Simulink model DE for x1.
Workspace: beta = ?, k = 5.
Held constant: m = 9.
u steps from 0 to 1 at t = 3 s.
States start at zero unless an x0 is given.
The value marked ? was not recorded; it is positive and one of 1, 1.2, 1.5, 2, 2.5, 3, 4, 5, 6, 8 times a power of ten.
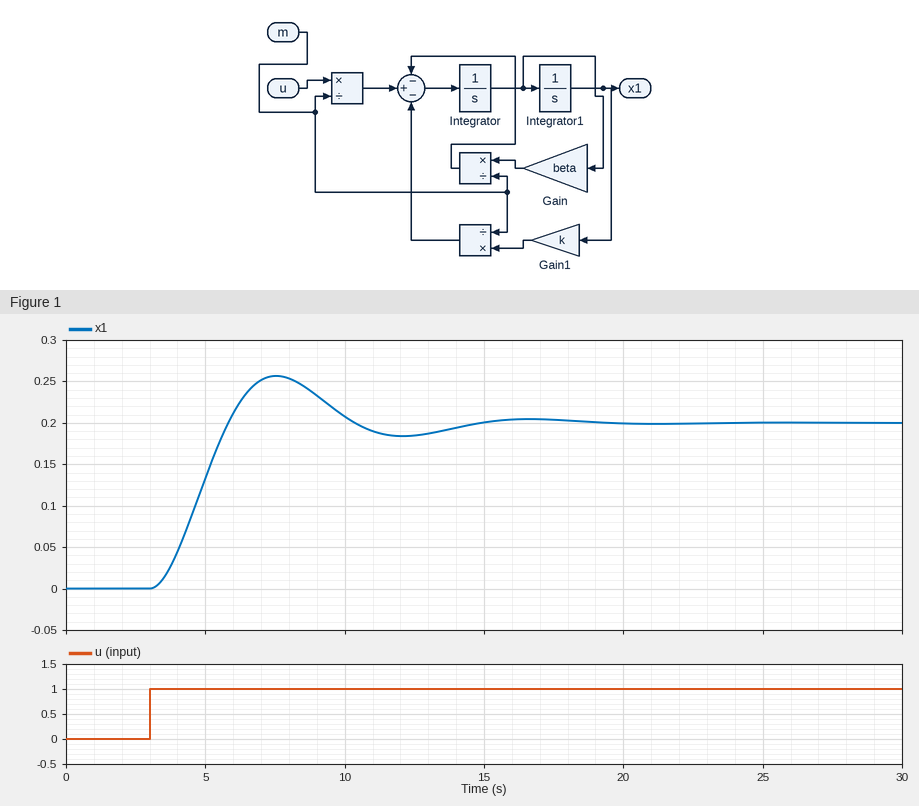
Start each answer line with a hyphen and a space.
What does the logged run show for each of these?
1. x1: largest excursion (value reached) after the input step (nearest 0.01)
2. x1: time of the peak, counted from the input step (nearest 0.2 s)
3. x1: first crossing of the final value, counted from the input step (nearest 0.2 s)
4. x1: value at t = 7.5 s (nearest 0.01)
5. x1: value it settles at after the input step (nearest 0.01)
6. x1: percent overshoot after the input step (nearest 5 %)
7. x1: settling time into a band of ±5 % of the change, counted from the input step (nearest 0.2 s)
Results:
- 0.26
- 4.6 s
- 2.8 s
- 0.26
- 0.20
- 30 %
- 10.4 s
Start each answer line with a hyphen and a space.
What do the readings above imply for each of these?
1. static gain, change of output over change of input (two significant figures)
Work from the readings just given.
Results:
- 0.20
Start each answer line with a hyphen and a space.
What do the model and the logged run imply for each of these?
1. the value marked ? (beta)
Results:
- 5
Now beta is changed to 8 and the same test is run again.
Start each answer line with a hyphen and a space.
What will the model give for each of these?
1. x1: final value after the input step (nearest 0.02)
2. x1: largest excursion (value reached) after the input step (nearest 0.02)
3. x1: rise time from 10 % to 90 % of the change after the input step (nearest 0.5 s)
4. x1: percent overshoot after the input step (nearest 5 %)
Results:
- 0.20
- 0.22
- 2.5 s
- 10 %
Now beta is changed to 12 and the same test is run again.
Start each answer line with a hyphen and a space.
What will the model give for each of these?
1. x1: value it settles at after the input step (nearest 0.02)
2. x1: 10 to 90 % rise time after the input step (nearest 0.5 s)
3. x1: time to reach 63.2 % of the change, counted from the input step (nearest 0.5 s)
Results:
- 0.20
- 4.0 s
- 2.5 s
